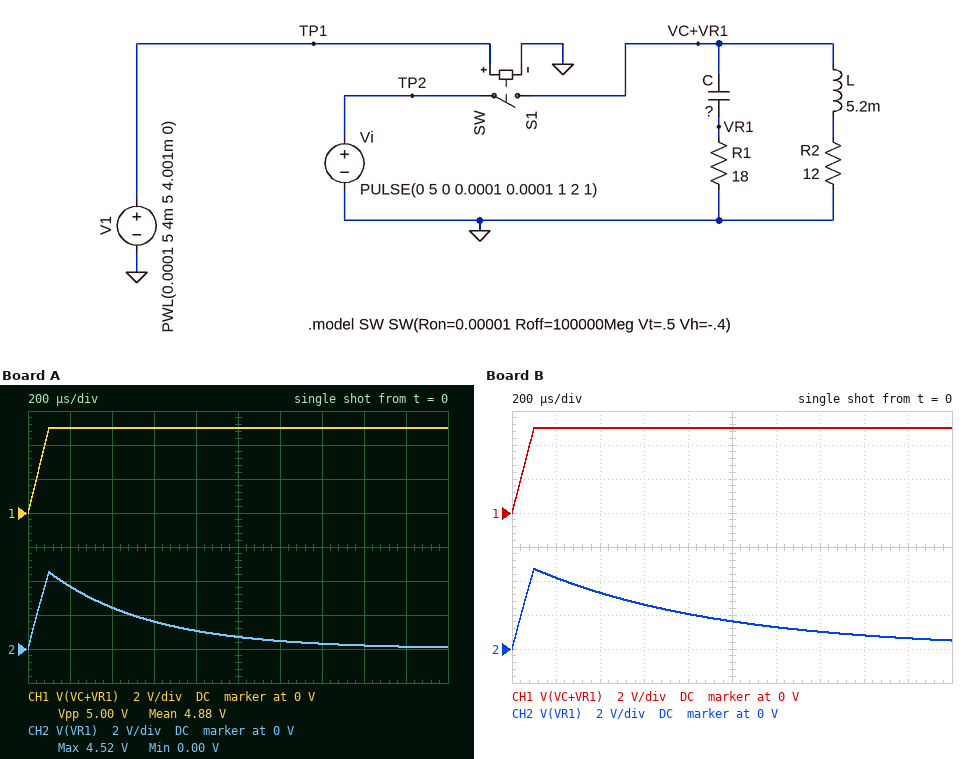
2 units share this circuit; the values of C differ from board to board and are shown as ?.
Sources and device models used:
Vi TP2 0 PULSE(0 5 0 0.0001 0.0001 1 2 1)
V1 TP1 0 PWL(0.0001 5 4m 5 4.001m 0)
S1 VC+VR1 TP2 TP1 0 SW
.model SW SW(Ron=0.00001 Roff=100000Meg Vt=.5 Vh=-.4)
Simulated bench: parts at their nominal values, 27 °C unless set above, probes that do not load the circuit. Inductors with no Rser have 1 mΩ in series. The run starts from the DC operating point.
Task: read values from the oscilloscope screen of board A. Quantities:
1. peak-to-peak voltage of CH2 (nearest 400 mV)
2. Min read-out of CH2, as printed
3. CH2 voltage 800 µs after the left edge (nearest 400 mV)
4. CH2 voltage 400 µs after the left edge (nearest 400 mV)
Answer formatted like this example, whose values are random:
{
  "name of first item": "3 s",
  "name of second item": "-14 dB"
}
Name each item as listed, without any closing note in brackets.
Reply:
{
  "peak-to-peak voltage of CH2": "4.4 V",
  "Min read-out of CH2, as printed": "0.00 V",
  "CH2 voltage 800 µs after the left edge": "1.2 V",
  "CH2 voltage 400 µs after the left edge": "2.4 V"
}
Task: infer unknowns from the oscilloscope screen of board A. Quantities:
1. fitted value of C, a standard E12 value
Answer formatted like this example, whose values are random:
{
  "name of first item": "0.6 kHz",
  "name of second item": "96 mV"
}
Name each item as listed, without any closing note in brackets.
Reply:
{
  "fitted value of C, a standard E12 value": "27 µF"
}
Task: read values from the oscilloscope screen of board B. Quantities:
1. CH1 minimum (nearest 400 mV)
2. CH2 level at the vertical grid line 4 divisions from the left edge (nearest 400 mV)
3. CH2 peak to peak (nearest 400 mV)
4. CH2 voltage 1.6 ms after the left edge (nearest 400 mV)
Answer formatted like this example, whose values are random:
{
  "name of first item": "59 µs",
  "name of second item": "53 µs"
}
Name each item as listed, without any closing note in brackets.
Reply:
{
  "CH1 minimum": "0 V",
  "CH2 level at the vertical grid line 4 divisions from the left edge": "2.0 V",
  "CH2 peak to peak": "4.8 V",
  "CH2 voltage 1.6 ms after the left edge": "800 mV"
}
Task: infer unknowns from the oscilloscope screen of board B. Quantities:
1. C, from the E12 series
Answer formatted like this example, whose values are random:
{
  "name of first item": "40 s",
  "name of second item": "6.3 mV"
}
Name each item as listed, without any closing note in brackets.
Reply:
{
  "C, from the E12 series": "47 µF"
}
